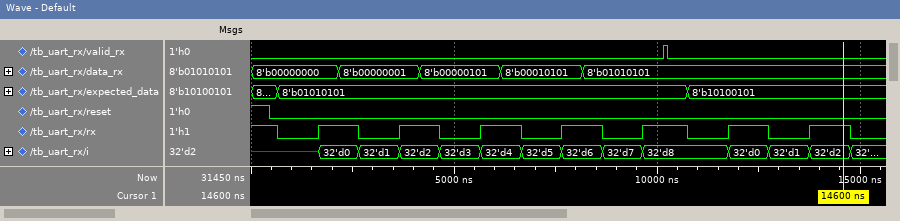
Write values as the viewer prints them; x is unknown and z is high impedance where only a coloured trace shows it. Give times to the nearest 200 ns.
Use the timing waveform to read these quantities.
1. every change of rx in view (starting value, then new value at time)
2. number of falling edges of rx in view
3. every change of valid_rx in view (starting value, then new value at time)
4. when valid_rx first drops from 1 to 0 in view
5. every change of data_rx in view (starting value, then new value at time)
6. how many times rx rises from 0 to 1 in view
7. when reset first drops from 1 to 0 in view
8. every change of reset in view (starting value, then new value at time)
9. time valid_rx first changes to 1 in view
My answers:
1, 0 at 600 ns, 1 at 1600 ns, 0 at 2600 ns, 1 at 3600 ns, 0 at 4600 ns, 1 at 5600 ns, 0 at 6600 ns, 1 at 7600 ns, 0 at 8600 ns, 1 at 9600 ns, 0 at 10800 ns, 1 at 11800 ns, 0 at 12800 ns, 1 at 13800 ns, 0 at 14800 ns
8
0, 1 at 10200 ns, 0 at 10200 ns
10200 ns
8'b00000000, 8'b00000001 at 2200 ns, 8'b00000101 at 4200 ns, 8'b00010101 at 6200 ns, 8'b01010101 at 8200 ns
7
400 ns
1, 0 at 400 ns
10200 ns
